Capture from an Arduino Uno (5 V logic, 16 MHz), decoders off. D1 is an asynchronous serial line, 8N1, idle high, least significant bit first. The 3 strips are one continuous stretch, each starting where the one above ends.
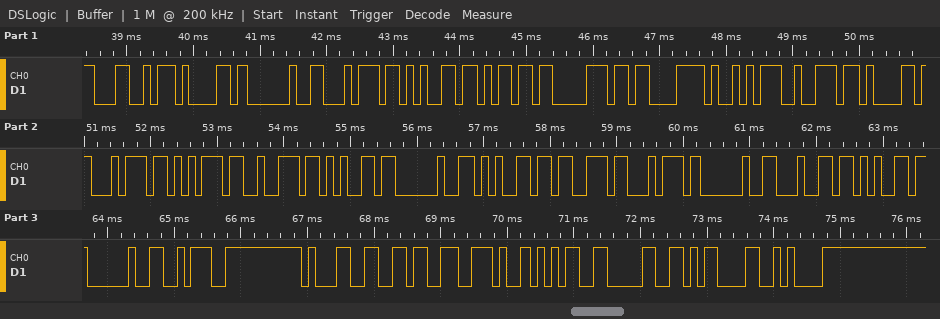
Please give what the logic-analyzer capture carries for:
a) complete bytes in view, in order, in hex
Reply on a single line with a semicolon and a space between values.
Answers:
4C 61 20 74 65 6D 70 C3 A9 72 61 74 75 72 65 20 65 73 74 20 64 65 20 3A 31 36 2E 35 30 0D 0A
